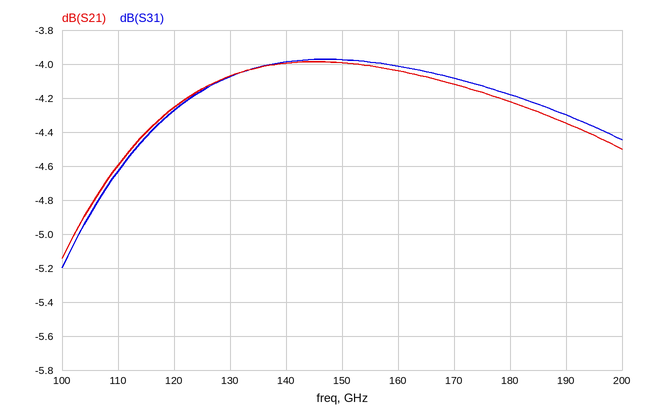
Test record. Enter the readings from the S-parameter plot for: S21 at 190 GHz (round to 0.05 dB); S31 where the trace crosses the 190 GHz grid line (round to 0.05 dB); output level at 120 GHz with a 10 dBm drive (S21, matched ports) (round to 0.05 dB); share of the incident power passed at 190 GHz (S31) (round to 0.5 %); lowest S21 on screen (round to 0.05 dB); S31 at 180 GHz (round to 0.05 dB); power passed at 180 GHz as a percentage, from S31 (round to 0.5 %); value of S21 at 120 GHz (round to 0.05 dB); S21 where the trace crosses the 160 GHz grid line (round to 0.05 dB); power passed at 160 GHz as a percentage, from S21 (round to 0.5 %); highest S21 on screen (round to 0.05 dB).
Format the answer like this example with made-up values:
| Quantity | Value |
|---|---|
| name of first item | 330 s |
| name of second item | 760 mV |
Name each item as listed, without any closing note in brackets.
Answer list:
| Quantity | Value |
|---|---|
| S21 at 190 GHz | -4.35 dB |
| S31 where the trace crosses the 190 GHz grid line | -4.30 dB |
| output level at 120 GHz with a 10 dBm drive (S21, matched ports) | 5.75 dBm |
| share of the incident power passed at 190 GHz (S31) | 37.0 % |
| lowest S21 on screen | -5.15 dB |
| S31 at 180 GHz | -4.20 dB |
| power passed at 180 GHz as a percentage, from S31 | 38.0 % |
| value of S21 at 120 GHz | -4.25 dB |
| S21 where the trace crosses the 160 GHz grid line | -4.05 dB |
| power passed at 160 GHz as a percentage, from S21 | 39.5 % |
| highest S21 on screen | -4.00 dB |
